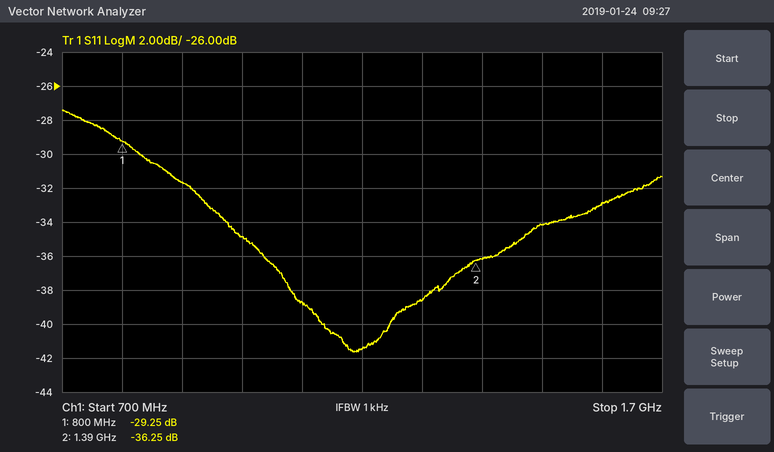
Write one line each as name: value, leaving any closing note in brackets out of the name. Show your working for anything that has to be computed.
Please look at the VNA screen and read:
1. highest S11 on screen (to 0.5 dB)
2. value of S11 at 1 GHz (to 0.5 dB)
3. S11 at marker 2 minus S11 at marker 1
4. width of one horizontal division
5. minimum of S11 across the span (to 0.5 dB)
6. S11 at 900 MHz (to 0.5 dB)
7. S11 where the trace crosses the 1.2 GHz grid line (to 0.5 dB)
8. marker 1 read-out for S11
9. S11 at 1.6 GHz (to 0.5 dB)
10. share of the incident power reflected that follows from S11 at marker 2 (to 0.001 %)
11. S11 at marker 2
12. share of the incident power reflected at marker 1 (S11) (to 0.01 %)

highest S11 on screen: -27.5 dB
value of S11 at 1 GHz: -35.0 dB
S11 at marker 2 minus S11 at marker 1: -36.25 − (-29.25) = -7.00 dB
width of one horizontal division: 100 MHz
minimum of S11 across the span: -41.5 dB
S11 at 900 MHz: -31.5 dB
S11 where the trace crosses the 1.2 GHz grid line: -41.5 dB
marker 1 read-out for S11: -29.25 dB
S11 at 1.6 GHz: -33.0 dB
share of the incident power reflected that follows from S11 at marker 2: 10^(-36.25/10) ≈ 0.024 %
S11 at marker 2: -36.25 dB
share of the incident power reflected at marker 1 (S11): 10^(-29.25/10) ≈ 0.12 %
